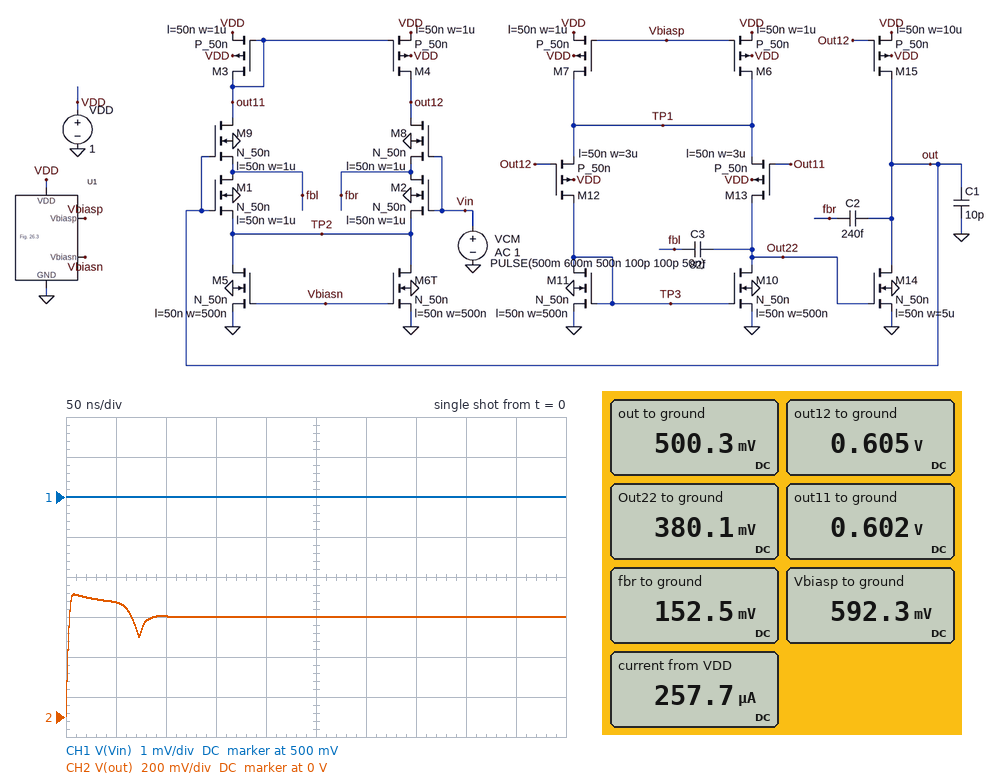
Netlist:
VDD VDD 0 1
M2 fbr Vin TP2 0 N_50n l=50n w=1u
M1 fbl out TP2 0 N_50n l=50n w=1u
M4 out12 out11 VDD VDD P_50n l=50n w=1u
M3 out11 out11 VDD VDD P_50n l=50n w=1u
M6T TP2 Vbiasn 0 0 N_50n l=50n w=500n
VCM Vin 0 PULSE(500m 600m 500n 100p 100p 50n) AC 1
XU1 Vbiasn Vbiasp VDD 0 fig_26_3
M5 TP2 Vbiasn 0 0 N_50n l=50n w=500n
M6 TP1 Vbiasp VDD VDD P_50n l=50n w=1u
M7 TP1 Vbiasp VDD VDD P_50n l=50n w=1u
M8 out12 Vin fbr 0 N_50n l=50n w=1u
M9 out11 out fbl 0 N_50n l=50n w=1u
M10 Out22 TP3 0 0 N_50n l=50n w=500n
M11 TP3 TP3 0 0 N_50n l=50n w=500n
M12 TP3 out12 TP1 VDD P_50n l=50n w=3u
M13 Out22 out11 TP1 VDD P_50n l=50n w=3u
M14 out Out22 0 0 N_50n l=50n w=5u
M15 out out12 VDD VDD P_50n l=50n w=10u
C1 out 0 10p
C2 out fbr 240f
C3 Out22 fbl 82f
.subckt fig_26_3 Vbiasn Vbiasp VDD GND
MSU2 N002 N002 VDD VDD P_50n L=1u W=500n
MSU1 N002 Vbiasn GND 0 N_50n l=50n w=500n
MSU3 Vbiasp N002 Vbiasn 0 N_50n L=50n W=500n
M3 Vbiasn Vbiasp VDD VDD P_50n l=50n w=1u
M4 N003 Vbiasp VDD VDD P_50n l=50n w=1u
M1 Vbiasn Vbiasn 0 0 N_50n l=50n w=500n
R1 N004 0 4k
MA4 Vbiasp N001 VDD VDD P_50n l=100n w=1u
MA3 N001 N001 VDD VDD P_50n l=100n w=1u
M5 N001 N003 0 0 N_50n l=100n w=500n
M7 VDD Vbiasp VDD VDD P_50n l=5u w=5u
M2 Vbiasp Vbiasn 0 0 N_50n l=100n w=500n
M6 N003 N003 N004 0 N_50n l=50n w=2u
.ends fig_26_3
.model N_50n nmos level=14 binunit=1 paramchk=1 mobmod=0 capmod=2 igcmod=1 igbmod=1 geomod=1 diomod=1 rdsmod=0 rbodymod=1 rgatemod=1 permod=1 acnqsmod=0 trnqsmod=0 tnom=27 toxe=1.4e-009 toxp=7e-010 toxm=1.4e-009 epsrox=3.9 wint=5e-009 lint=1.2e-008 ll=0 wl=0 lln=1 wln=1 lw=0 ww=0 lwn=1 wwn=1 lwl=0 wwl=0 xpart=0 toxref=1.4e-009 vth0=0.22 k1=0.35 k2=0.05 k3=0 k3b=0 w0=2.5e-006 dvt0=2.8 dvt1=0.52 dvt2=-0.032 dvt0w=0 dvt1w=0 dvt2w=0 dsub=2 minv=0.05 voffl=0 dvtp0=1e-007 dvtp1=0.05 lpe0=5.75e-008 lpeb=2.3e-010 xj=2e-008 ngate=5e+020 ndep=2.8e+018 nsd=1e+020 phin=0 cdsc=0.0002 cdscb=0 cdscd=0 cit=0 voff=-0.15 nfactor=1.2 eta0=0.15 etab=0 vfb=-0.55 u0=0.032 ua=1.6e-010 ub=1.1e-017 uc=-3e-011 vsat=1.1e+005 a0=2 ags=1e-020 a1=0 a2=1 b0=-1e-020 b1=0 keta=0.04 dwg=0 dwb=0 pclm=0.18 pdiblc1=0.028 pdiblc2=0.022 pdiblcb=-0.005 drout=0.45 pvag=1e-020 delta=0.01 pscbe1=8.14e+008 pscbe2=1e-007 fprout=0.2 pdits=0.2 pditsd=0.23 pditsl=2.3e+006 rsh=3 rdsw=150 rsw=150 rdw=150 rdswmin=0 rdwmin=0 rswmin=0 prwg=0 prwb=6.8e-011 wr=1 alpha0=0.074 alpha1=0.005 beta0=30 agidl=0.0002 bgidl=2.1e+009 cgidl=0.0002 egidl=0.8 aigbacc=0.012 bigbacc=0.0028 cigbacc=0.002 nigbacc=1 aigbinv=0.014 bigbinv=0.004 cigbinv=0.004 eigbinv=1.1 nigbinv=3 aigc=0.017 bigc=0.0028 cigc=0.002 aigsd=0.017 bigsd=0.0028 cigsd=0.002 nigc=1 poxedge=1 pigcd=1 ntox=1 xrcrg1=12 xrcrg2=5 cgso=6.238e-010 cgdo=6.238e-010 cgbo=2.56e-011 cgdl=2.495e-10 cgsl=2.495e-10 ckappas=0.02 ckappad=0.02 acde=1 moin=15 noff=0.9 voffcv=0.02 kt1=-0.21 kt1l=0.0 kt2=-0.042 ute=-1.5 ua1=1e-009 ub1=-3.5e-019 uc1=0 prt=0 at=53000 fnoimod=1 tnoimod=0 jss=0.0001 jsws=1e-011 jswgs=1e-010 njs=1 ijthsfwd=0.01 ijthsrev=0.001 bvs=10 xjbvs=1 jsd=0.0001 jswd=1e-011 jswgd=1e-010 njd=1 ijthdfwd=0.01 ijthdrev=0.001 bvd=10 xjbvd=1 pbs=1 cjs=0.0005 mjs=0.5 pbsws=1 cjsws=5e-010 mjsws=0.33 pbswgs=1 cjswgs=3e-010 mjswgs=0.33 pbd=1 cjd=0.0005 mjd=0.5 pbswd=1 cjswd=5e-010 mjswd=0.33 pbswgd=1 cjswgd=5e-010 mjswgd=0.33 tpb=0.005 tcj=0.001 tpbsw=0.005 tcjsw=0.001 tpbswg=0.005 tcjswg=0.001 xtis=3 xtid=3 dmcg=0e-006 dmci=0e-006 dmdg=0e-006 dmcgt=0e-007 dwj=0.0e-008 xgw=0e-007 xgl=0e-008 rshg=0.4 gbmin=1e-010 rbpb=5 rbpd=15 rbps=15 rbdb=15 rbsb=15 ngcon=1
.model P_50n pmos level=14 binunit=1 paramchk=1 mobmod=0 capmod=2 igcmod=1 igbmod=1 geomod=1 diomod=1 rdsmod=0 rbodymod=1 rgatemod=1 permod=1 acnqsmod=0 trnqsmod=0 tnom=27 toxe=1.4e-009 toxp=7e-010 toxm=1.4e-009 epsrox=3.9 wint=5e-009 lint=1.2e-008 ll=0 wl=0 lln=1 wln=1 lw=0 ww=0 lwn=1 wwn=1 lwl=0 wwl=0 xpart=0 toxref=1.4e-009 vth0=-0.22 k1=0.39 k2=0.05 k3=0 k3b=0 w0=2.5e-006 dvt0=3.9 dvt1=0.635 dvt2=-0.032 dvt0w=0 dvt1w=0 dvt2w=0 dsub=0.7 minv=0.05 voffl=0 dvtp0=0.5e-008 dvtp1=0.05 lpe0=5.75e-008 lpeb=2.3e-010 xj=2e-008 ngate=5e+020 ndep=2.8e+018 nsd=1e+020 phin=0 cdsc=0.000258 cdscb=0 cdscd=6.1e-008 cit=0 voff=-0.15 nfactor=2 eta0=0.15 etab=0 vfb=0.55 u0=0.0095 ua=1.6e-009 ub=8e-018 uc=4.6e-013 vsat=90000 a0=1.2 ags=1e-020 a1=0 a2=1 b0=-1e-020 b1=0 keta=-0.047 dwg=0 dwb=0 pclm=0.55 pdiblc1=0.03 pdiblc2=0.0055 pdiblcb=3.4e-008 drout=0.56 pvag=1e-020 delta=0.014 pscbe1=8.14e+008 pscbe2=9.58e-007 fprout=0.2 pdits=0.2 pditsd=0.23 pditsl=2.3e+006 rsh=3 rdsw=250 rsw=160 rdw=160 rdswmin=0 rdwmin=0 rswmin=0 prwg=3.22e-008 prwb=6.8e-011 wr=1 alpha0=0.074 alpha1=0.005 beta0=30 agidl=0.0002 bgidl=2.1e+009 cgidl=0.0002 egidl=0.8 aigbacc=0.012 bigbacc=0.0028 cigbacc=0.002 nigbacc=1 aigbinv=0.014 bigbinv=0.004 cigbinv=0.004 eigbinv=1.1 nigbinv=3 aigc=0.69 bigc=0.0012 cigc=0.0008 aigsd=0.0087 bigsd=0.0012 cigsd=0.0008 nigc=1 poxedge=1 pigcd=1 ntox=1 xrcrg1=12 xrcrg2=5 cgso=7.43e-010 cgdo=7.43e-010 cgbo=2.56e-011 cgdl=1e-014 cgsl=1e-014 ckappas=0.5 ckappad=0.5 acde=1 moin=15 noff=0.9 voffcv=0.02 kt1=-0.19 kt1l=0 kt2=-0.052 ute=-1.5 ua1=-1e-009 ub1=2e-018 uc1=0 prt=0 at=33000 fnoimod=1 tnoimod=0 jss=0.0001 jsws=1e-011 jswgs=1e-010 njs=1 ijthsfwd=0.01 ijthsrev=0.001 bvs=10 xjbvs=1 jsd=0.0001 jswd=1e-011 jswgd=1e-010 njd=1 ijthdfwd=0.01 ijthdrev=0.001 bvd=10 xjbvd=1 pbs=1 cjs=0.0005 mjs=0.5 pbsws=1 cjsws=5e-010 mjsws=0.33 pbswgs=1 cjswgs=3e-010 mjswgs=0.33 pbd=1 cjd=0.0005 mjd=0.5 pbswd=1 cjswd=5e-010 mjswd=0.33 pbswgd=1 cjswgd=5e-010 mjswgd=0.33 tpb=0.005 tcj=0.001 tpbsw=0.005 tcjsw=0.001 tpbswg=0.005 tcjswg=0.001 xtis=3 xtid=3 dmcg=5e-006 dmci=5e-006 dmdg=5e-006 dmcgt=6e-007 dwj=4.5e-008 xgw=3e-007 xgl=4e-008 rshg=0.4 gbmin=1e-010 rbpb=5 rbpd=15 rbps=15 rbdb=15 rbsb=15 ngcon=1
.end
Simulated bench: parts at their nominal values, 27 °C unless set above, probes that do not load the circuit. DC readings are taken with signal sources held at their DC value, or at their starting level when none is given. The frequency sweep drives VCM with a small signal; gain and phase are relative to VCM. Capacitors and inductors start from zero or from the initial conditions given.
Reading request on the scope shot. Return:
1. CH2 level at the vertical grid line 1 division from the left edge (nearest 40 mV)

560 mV
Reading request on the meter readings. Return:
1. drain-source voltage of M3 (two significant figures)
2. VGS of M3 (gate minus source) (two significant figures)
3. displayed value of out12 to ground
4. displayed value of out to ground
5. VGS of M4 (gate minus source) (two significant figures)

-400 mV
-400 mV
0.605 V
500.3 mV
-400 mV
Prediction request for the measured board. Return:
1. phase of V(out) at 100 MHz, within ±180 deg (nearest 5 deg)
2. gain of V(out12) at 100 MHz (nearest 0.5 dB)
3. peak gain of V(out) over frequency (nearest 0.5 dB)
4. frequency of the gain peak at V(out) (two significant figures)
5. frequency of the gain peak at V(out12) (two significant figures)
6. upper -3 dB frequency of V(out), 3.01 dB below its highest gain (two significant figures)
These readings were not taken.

-35 deg
5.0 dB
3.5 dB
130 MHz
180 MHz
190 MHz
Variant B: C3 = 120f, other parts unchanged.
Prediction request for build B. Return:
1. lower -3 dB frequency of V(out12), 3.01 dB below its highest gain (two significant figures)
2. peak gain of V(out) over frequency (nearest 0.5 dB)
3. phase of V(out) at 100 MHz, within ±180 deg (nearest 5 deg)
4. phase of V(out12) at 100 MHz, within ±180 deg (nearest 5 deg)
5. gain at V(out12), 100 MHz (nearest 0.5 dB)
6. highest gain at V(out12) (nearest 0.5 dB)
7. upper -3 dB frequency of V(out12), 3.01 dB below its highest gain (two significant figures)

100 MHz
2.0 dB
-45 deg
-105 deg
6.5 dB
10.0 dB
520 MHz
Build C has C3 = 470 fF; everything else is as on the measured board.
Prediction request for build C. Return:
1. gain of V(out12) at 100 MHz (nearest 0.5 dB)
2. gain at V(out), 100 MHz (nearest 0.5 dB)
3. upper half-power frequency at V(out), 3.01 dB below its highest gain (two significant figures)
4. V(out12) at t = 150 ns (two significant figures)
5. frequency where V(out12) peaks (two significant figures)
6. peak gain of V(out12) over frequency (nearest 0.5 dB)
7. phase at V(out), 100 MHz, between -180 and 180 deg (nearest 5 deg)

5.5 dB
-2.5 dB
110 MHz
670 mV
280 MHz
7.5 dB
-55 deg
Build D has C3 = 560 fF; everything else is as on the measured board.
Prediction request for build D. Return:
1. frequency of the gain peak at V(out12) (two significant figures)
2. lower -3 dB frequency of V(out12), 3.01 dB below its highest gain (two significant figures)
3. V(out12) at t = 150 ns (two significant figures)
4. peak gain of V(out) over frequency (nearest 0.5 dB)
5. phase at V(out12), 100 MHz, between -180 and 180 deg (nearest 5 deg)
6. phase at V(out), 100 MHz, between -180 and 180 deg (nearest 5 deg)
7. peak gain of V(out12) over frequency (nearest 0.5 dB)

290 MHz
89 MHz
670 mV
0 dB
-145 deg
-55 deg
7.5 dB
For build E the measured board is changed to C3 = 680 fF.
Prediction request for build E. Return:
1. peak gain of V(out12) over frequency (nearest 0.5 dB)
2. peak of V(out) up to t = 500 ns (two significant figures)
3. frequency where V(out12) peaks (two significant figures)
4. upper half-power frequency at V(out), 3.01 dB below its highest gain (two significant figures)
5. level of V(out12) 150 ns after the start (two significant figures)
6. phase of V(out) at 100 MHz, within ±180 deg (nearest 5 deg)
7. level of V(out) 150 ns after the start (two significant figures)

7.5 dB
590 mV
290 MHz
94 MHz
680 mV
-55 deg
510 mV
